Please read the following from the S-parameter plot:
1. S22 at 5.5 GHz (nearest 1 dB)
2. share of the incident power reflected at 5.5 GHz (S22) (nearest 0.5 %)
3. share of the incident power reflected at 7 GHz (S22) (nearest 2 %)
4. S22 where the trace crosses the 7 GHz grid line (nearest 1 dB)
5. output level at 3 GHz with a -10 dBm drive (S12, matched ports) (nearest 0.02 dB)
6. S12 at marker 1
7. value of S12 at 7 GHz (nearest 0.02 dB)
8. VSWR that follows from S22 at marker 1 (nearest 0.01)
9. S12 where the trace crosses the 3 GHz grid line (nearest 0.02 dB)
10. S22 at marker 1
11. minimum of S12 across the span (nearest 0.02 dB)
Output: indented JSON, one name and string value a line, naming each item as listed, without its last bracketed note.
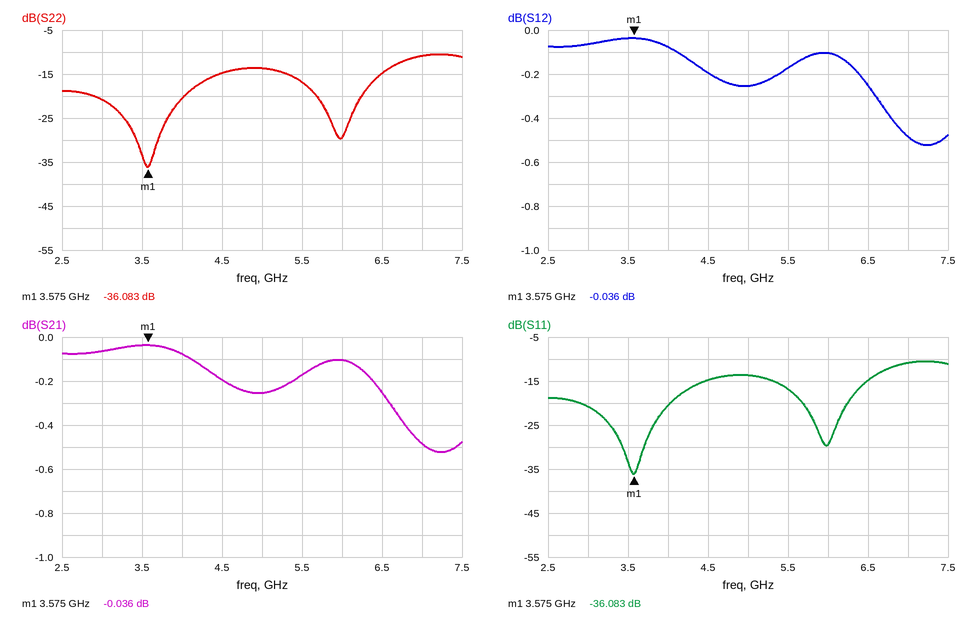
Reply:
{
  "S22 at 5.5 GHz": "-17 dB",
  "share of the incident power reflected at 5.5 GHz (S22)": "2.0 %",
  "share of the incident power reflected at 7 GHz (S22)": "8 %",
  "S22 where the trace crosses the 7 GHz grid line": "-11 dB",
  "output level at 3 GHz with a -10 dBm drive (S12, matched ports)": "-10.06 dBm",
  "S12 at marker 1": "-0.036 dB",
  "value of S12 at 7 GHz": "-0.48 dB",
  "VSWR that follows from S22 at marker 1": "1.03",
  "S12 where the trace crosses the 3 GHz grid line": "-0.06 dB",
  "S22 at marker 1": "-36.083 dB",
  "minimum of S12 across the span": "-0.52 dB"
}
